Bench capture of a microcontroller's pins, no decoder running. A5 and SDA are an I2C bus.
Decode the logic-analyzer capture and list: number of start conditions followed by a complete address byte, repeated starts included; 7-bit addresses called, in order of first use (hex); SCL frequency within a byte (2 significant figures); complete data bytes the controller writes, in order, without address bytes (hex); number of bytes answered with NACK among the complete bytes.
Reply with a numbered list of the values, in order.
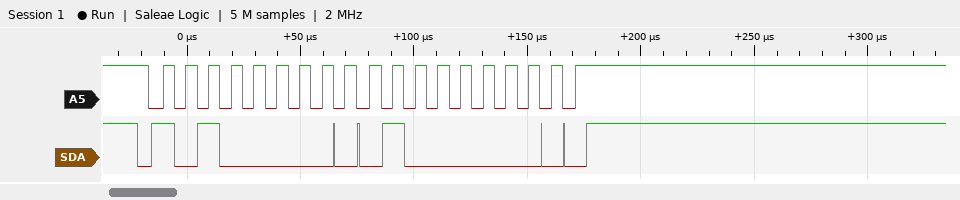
1. 1
2. 0x50
3. 100 kHz
4. 40
5. 0
